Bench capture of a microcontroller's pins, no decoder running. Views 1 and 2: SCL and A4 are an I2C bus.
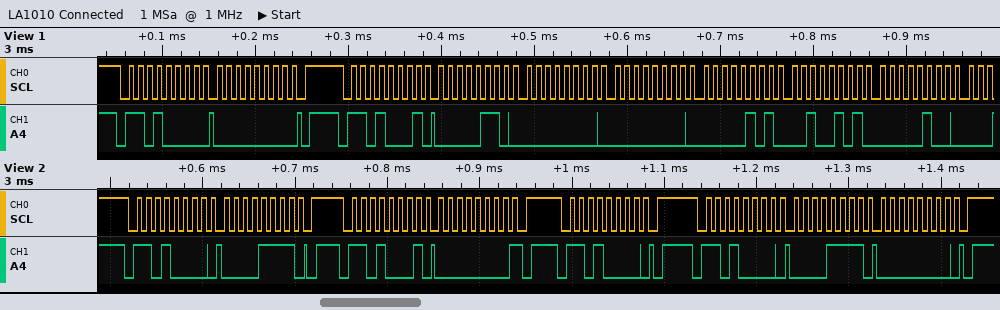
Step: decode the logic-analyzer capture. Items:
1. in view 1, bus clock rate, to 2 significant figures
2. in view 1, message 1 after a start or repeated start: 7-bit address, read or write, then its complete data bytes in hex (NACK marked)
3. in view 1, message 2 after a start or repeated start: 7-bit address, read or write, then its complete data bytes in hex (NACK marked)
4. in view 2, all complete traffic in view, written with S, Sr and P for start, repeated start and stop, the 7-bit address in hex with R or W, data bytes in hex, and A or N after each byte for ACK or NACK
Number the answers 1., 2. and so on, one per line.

1. 100 kHz
2. 0x68 write: 00
3. 0x68 read: 06 00 00 05 25 04
4. S 68W A 0F A P S 68R A 00 N P S 68W A P S 68W A 0F A 00 A P
